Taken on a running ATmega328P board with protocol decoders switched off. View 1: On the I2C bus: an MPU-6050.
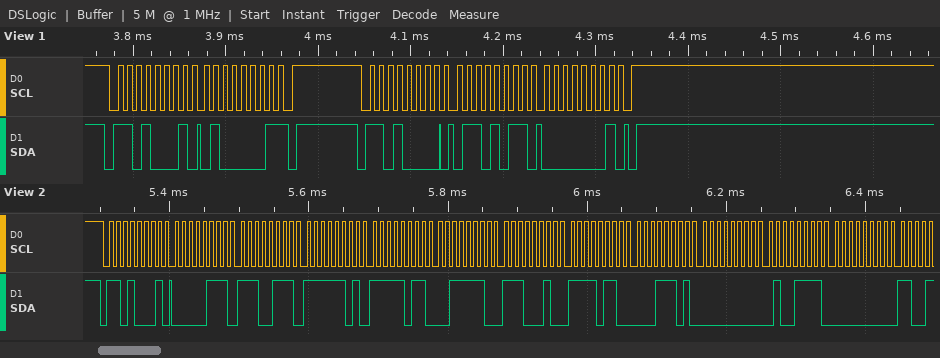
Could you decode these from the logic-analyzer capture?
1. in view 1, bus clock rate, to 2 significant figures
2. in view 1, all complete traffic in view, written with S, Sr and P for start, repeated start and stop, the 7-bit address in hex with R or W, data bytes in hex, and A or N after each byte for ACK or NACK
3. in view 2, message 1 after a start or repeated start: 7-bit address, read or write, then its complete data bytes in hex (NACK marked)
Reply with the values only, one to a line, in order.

100 kHz
S 68R A 41 N P S 68W A 6B A 01 A P
0x68 read: 07 E7 FD FB 3E E2 F6 1D 00 4F 00
